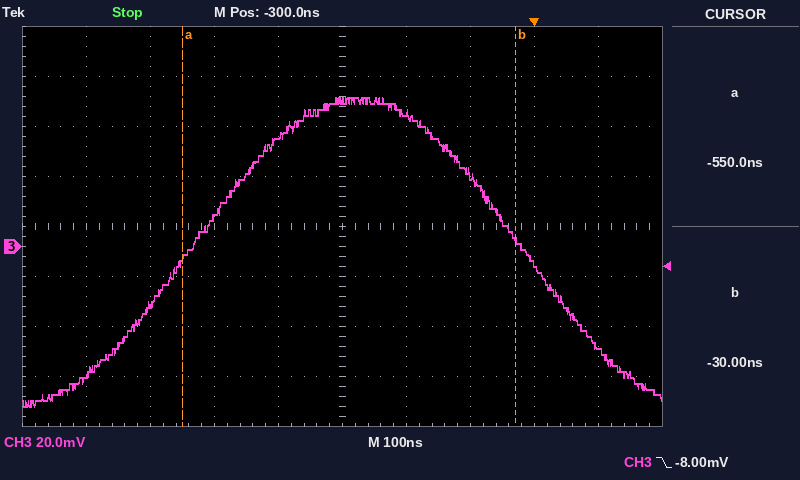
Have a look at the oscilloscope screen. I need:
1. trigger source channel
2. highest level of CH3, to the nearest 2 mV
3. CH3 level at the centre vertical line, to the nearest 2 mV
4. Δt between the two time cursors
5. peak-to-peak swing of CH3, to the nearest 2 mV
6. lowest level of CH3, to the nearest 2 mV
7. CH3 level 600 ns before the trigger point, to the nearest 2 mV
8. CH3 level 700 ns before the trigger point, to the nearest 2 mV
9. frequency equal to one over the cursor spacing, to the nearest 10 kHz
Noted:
CH3
60 mV
58 mV
520 ns
124 mV
-64 mV
-24 mV
-52 mV
1.92 MHz
